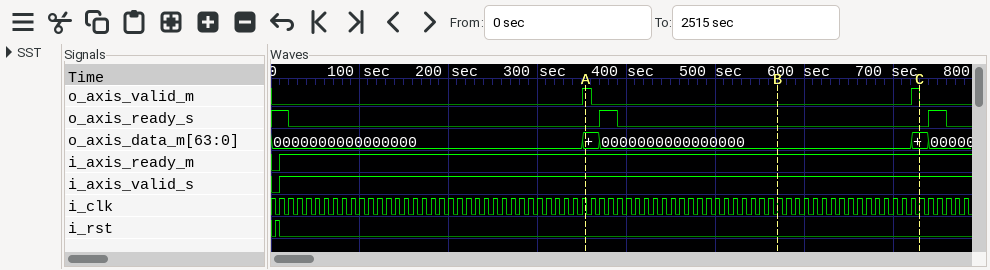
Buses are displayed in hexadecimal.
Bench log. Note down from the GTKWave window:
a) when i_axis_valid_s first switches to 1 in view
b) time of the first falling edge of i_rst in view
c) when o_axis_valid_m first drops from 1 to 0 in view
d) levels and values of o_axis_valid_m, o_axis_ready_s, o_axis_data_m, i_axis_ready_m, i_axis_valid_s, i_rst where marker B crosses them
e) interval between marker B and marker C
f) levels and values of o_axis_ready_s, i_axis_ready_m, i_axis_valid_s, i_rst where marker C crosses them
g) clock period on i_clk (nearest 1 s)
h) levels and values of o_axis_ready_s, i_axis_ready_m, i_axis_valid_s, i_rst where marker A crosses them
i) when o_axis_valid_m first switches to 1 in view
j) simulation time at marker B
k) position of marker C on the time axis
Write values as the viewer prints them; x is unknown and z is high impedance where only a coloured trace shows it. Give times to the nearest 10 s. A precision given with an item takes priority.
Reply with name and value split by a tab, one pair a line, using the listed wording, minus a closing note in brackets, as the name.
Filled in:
when i_axis_valid_s first switches to 1 in view	10 s
time of the first falling edge of i_rst in view	10 s
when o_axis_valid_m first drops from 1 to 0 in view	360 s
levels and values of o_axis_valid_m, o_axis_ready_s, o_axis_data_m, i_axis_ready_m, i_axis_valid_s, i_rst where marker B crosses them	o_axis_valid_m=0, o_axis_ready_s=0, o_axis_data_m=0000000000000000, i_axis_ready_m=1, i_axis_valid_s=1, i_rst=0
interval between marker B and marker C	160 s
levels and values of o_axis_ready_s, i_axis_ready_m, i_axis_valid_s, i_rst where marker C crosses them	o_axis_ready_s=0, i_axis_ready_m=1, i_axis_valid_s=1, i_rst=0
clock period on i_clk	10 s
levels and values of o_axis_ready_s, i_axis_ready_m, i_axis_valid_s, i_rst where marker A crosses them	o_axis_ready_s=0, i_axis_ready_m=1, i_axis_valid_s=1, i_rst=0
when o_axis_valid_m first switches to 1 in view	350 s
simulation time at marker B	570 s
position of marker C on the time axis	730 s
